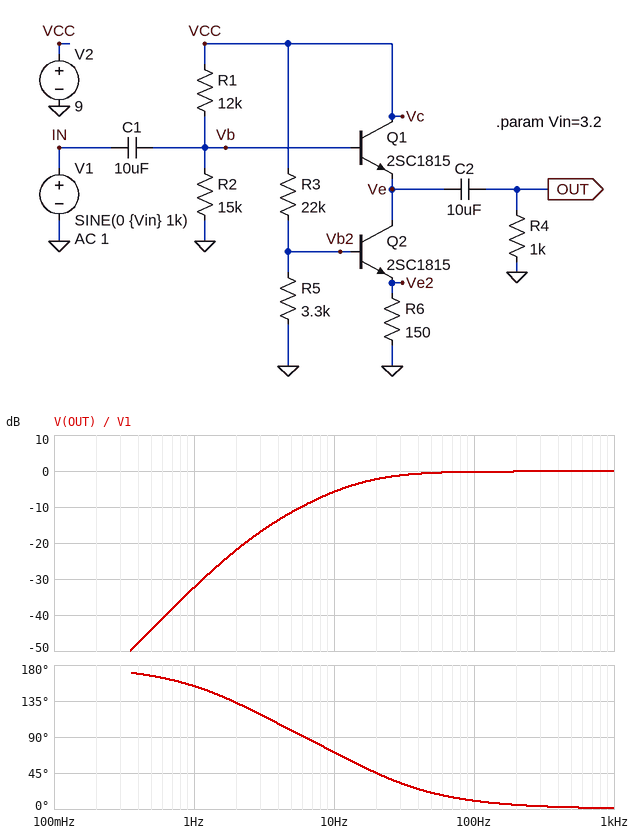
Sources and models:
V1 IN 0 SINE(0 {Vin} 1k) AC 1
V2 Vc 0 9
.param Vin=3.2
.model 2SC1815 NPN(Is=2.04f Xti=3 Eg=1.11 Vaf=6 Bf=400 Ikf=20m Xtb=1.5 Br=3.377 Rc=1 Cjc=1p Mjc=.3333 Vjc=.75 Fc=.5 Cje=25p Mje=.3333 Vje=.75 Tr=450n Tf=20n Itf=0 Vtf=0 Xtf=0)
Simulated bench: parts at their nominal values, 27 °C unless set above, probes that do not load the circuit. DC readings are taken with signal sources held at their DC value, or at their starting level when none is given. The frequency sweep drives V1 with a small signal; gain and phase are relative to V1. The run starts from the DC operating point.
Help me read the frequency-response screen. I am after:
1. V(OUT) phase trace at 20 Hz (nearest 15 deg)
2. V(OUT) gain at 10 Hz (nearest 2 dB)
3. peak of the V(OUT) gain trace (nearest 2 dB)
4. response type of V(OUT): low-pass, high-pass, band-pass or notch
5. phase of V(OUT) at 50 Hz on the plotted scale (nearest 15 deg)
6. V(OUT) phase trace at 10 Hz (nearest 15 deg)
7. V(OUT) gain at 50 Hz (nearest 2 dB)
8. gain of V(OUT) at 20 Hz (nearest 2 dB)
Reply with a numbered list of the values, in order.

1. 45 deg
2. -6 dB
3. 0 dB
4. high-pass
5. 15 deg
6. 75 deg
7. 0 dB
8. -2 dB
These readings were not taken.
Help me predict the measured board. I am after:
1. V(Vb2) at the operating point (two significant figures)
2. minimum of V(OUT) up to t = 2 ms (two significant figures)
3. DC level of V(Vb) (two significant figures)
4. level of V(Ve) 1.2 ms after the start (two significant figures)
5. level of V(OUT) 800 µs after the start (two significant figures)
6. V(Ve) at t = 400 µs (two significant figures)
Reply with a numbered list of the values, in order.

1. 1.2 V
2. -2.8 V
3. 5.0 V
4. 7.3 V
5. -2.8 V
6. 6.1 V
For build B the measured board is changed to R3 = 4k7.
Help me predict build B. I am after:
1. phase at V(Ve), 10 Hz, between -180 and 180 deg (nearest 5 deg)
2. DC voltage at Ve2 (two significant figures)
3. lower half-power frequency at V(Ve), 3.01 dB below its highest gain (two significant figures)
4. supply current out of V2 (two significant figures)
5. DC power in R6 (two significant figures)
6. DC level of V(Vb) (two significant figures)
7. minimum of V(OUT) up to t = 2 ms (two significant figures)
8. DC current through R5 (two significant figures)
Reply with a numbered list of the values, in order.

1. 15 deg
2. 2.8 V
3. 2.5 Hz
4. 20 mA
5. 51 mW
6. 4.7 V
7. -3.2 V
8. 1.1 mA
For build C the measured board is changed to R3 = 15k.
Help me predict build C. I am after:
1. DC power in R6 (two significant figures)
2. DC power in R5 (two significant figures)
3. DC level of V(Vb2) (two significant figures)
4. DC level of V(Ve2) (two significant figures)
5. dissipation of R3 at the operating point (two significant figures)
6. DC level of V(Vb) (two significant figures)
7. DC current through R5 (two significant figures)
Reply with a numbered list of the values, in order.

1. 4.9 mW
2. 770 µW
3. 1.6 V
4. 850 mV
5. 3.7 mW
6. 4.9 V
7. 480 µA
